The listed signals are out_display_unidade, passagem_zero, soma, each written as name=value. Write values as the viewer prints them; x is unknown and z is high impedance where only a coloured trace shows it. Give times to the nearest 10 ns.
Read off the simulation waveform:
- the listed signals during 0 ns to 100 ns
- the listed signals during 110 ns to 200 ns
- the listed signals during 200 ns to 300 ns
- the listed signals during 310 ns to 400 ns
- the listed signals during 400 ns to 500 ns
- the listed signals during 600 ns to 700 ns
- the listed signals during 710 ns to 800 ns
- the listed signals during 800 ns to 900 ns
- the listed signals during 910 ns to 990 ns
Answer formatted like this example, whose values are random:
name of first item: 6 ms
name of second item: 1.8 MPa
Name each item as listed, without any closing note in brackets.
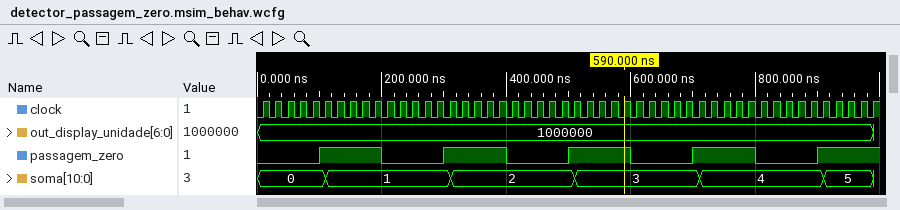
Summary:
the listed signals during 0 ns to 100 ns: out_display_unidade=1000000, passagem_zero=0, soma=0
the listed signals during 110 ns to 200 ns: out_display_unidade=1000000, passagem_zero=1, soma=1
the listed signals during 200 ns to 300 ns: out_display_unidade=1000000, passagem_zero=0, soma=1
the listed signals during 310 ns to 400 ns: out_display_unidade=1000000, passagem_zero=1, soma=2
the listed signals during 400 ns to 500 ns: out_display_unidade=1000000, passagem_zero=0, soma=2
the listed signals during 600 ns to 700 ns: out_display_unidade=1000000, passagem_zero=0, soma=3
the listed signals during 710 ns to 800 ns: out_display_unidade=1000000, passagem_zero=1, soma=4
the listed signals during 800 ns to 900 ns: out_display_unidade=1000000, passagem_zero=0, soma=4
the listed signals during 910 ns to 990 ns: out_display_unidade=1000000, passagem_zero=1, soma=5
